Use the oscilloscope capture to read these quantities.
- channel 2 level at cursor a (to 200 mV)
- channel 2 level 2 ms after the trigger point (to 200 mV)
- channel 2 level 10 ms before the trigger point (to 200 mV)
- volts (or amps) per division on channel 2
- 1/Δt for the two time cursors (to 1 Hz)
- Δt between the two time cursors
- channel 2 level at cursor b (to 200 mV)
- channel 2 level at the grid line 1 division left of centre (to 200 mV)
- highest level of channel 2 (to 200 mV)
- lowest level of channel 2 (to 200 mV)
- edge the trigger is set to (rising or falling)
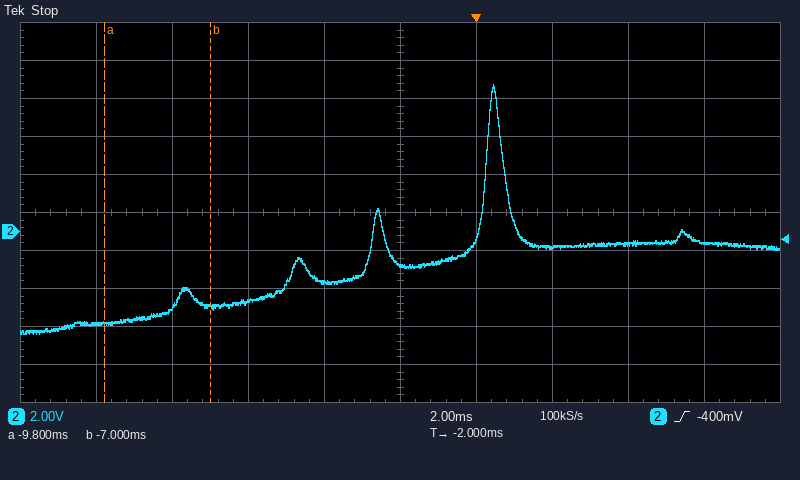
-4.8 V
-800 mV
-4.8 V
2 V
357 Hz
2.8 ms
-4.0 V
-2.6 V
7.8 V
-5.4 V
rising
